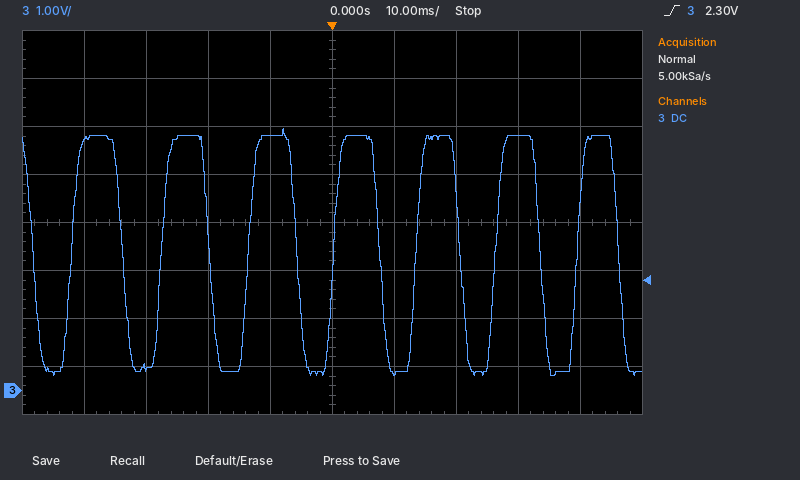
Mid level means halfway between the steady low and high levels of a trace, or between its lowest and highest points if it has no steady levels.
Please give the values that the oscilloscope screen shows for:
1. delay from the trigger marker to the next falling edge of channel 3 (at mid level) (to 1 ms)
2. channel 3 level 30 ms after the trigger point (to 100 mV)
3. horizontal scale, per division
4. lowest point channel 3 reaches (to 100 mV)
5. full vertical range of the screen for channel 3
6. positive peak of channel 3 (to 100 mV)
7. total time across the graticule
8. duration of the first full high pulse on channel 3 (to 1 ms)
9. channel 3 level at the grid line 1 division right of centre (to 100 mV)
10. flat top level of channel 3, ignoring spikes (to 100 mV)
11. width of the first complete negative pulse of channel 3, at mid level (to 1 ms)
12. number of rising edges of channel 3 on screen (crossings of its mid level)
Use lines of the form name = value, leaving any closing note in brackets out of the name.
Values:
delay from the trigger marker to the next falling edge of channel 3 (at mid level) = 8 ms
channel 3 level 30 ms after the trigger point = 5.3 V
horizontal scale, per division = 10 ms
lowest point channel 3 reaches = 300 mV
full vertical range of the screen for channel 3 = 8 V
positive peak of channel 3 = 5.5 V
total time across the graticule = 100 ms
duration of the first full high pulse on channel 3 = 8 ms
channel 3 level at the grid line 1 division right of centre = 400 mV
flat top level of channel 3, ignoring spikes = 5.3 V
width of the first complete negative pulse of channel 3, at mid level = 6 ms
number of rising edges of channel 3 on screen = 7
